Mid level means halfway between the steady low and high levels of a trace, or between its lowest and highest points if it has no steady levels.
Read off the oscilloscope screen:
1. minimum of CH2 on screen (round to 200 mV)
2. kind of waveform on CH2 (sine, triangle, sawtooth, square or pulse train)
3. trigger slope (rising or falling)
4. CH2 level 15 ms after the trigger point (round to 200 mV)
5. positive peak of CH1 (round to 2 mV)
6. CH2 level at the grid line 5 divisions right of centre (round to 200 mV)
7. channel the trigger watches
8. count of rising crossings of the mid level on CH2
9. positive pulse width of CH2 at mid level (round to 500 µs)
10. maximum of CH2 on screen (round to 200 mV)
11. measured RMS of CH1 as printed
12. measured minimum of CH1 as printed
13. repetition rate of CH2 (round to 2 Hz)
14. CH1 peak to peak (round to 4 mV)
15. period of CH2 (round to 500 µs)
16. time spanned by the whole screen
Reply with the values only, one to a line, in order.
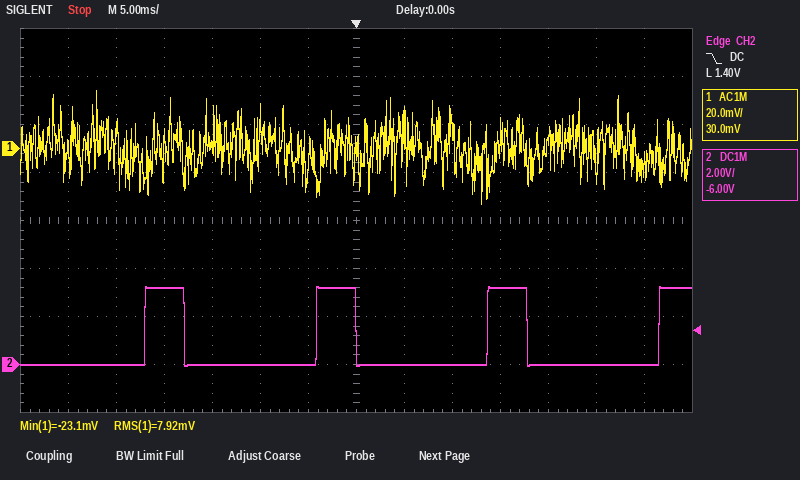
0.0 V
pulse train
falling
3.2 V
24 mV
0.0 V
CH2
4
4.0 ms
3.2 V
7.92 mV
-23.1 mV
56 Hz
48 mV
18.0 ms
70 ms
